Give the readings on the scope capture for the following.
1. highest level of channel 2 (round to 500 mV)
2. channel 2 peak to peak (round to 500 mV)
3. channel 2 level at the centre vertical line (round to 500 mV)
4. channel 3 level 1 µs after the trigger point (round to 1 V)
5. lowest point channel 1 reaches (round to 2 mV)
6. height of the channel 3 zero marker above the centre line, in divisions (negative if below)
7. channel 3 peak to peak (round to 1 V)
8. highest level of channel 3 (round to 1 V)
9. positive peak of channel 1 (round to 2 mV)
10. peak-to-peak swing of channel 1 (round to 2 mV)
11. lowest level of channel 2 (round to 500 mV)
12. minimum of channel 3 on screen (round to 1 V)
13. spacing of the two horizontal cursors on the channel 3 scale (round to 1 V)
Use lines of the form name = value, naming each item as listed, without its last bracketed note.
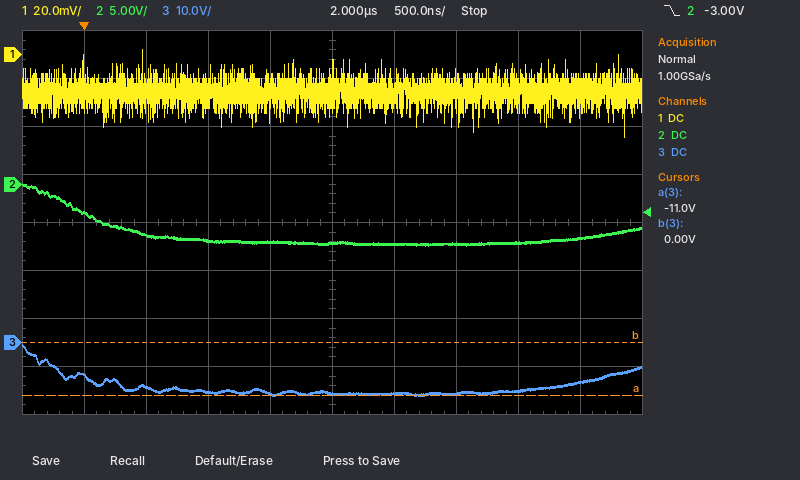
highest level of channel 2 = 0.0 V
channel 2 peak to peak = 6.5 V
channel 2 level at the centre vertical line = -6.0 V
channel 3 level 1 µs after the trigger point = -10 V
lowest point channel 1 reaches = -34 mV
height of the channel 3 zero marker above the centre line, in divisions = -2.5 div
channel 3 peak to peak = 11 V
highest level of channel 3 = 0 V
positive peak of channel 1 = 2 mV
peak-to-peak swing of channel 1 = 36 mV
lowest level of channel 2 = -6.5 V
minimum of channel 3 on screen = -11 V
spacing of the two horizontal cursors on the channel 3 scale = 11 V
